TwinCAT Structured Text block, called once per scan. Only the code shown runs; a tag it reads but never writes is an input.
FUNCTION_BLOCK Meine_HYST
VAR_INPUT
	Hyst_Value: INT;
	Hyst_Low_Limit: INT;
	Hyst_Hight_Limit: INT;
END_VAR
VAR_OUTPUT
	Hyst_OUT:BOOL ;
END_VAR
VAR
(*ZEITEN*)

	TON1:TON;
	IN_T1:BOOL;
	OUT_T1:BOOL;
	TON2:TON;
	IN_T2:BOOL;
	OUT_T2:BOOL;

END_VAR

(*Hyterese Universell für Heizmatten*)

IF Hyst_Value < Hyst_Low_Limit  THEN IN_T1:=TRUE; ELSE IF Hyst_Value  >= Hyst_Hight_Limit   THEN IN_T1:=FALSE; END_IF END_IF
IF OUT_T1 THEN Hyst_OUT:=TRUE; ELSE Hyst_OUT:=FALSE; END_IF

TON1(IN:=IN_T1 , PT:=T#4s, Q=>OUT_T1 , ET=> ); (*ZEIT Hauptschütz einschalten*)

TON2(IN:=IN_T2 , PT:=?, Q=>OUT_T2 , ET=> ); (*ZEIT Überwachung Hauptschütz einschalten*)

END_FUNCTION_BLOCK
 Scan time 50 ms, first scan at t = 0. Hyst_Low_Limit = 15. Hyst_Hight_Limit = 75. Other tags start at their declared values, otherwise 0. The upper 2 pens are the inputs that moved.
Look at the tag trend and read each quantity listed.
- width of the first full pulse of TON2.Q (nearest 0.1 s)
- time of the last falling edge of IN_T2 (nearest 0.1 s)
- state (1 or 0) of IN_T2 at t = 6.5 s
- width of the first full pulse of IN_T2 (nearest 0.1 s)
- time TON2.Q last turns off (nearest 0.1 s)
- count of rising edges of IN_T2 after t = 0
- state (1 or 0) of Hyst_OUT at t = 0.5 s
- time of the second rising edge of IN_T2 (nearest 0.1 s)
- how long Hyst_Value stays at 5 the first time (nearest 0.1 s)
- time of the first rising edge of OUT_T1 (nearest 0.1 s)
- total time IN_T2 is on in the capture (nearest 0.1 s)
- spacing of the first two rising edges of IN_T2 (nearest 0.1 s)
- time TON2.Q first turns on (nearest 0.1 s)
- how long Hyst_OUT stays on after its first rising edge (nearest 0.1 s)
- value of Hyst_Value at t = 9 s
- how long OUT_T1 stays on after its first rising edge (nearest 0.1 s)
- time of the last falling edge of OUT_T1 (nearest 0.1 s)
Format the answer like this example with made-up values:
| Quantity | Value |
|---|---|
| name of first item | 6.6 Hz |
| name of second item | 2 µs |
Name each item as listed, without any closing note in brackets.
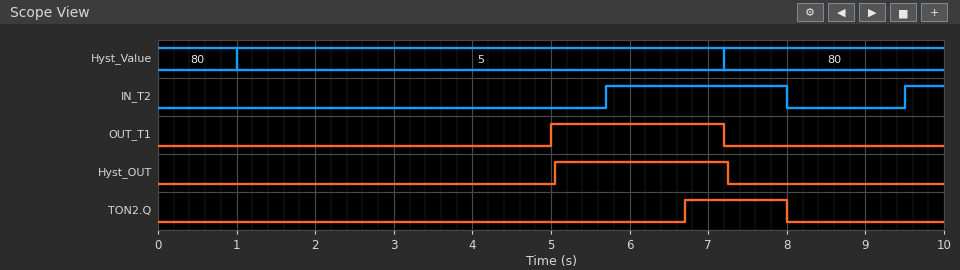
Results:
| Quantity | Value |
|---|---|
| width of the first full pulse of TON2.Q | 1.3 s |
| time of the last falling edge of IN_T2 | 8.0 s |
| state (1 or 0) of IN_T2 at t = 6.5 s | 1 |
| width of the first full pulse of IN_T2 | 2.3 s |
| time TON2.Q last turns off | 8.0 s |
| count of rising edges of IN_T2 after t = 0 | 2 |
| state (1 or 0) of Hyst_OUT at t = 0.5 s | 0 |
| time of the second rising edge of IN_T2 | 9.5 s |
| how long Hyst_Value stays at 5 the first time | 6.2 s |
| time of the first rising edge of OUT_T1 | 5.0 s |
| total time IN_T2 is on in the capture | 2.8 s |
| spacing of the first two rising edges of IN_T2 | 3.8 s |
| time TON2.Q first turns on | 6.7 s |
| how long Hyst_OUT stays on after its first rising edge | 2.2 s |
| value of Hyst_Value at t = 9 s | 80 |
| how long OUT_T1 stays on after its first rising edge | 2.2 s |
| time of the last falling edge of OUT_T1 | 7.2 s |
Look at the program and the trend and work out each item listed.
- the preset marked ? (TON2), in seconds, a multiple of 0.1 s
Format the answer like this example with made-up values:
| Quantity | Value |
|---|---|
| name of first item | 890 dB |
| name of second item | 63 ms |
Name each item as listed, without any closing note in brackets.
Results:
| Quantity | Value |
|---|---|
| the preset marked ? (TON2), in seconds, a multiple of 0.1 s | 1.0 s |
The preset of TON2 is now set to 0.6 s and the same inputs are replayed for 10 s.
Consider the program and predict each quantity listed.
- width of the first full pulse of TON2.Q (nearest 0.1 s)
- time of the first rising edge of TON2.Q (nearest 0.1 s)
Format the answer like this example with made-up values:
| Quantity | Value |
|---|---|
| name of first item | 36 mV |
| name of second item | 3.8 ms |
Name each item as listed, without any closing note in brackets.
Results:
| Quantity | Value |
|---|---|
| width of the first full pulse of TON2.Q | 1.7 s |
| time of the first rising edge of TON2.Q | 6.3 s |
